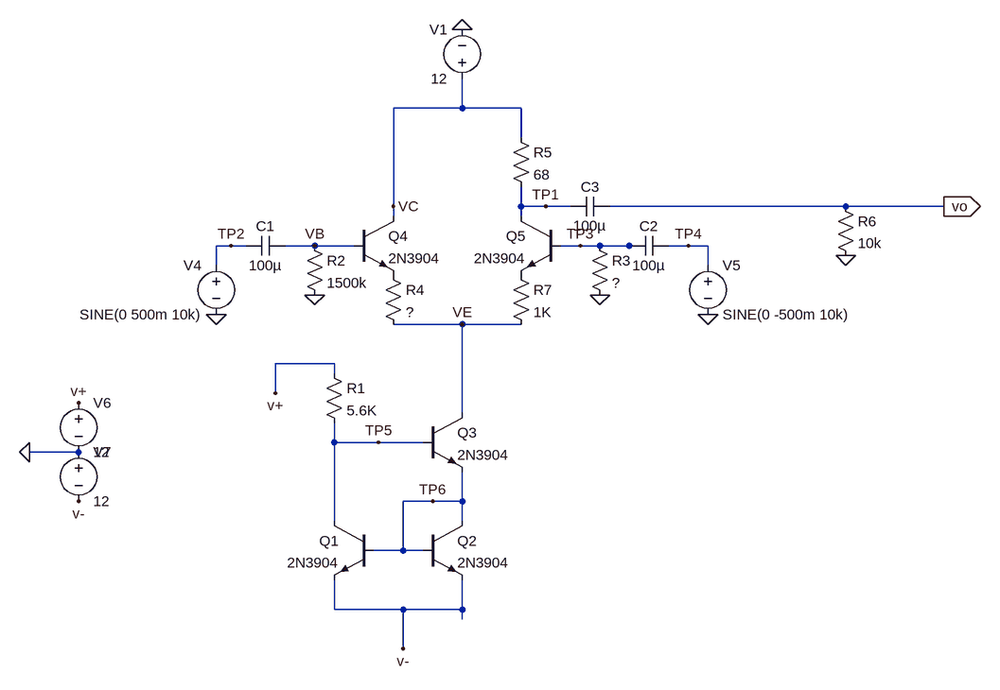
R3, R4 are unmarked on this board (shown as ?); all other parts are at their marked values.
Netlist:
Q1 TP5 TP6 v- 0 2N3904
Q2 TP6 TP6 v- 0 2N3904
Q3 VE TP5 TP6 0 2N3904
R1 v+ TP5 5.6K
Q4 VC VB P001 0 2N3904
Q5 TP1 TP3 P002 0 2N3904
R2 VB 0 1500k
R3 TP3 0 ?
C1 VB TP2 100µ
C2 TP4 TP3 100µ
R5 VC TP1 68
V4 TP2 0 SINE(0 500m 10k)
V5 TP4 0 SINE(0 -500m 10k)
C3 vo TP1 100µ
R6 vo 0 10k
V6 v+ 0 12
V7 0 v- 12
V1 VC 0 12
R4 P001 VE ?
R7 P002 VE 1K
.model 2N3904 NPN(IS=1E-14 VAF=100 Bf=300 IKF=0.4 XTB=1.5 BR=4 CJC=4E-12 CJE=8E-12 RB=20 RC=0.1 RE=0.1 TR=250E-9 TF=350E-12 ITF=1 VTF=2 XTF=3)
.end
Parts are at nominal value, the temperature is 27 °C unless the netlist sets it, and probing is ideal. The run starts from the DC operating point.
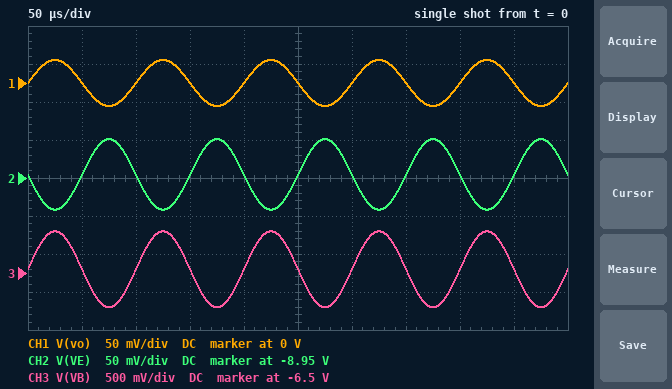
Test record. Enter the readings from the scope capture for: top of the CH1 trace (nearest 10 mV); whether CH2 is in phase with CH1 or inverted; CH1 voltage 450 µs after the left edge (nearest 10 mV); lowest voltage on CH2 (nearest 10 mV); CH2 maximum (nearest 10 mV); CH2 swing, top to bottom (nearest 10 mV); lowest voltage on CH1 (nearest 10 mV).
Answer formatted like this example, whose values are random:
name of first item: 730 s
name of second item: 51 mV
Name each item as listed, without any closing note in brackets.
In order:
top of the CH1 trace: 30 mV
whether CH2 is in phase with CH1 or inverted: inverted
CH1 voltage 450 µs after the left edge: 0 V
lowest voltage on CH2: -8.99 V
CH2 maximum: -8.90 V
CH2 swing, top to bottom: 90 mV
lowest voltage on CH1: -30 mV
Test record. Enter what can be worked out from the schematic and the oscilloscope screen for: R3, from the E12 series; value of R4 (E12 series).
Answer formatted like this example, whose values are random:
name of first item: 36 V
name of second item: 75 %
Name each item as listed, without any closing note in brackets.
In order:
R3, from the E12 series: 820 kΩ
value of R4: 1.2 kΩ
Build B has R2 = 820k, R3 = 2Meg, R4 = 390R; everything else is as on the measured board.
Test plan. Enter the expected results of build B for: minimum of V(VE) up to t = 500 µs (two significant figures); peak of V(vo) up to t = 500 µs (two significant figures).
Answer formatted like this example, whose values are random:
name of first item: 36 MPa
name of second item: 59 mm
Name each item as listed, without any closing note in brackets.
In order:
minimum of V(VE) up to t = 500 µs: -8.6 V
peak of V(vo) up to t = 500 µs: 47 mV
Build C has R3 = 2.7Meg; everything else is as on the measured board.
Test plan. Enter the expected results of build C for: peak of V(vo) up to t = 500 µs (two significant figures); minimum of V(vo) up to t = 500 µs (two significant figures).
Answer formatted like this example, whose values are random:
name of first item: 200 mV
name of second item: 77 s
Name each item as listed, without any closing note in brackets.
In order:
peak of V(vo) up to t = 500 µs: 33 mV
minimum of V(vo) up to t = 500 µs: -33 mV
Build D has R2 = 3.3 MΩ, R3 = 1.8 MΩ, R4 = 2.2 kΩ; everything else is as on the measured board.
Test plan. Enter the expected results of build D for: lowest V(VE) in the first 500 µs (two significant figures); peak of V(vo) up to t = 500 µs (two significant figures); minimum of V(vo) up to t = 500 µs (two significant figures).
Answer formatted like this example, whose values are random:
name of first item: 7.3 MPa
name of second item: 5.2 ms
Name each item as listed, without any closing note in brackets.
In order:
lowest V(VE) in the first 500 µs: -11 V
peak of V(vo) up to t = 500 µs: 33 mV
minimum of V(vo) up to t = 500 µs: -33 mV
